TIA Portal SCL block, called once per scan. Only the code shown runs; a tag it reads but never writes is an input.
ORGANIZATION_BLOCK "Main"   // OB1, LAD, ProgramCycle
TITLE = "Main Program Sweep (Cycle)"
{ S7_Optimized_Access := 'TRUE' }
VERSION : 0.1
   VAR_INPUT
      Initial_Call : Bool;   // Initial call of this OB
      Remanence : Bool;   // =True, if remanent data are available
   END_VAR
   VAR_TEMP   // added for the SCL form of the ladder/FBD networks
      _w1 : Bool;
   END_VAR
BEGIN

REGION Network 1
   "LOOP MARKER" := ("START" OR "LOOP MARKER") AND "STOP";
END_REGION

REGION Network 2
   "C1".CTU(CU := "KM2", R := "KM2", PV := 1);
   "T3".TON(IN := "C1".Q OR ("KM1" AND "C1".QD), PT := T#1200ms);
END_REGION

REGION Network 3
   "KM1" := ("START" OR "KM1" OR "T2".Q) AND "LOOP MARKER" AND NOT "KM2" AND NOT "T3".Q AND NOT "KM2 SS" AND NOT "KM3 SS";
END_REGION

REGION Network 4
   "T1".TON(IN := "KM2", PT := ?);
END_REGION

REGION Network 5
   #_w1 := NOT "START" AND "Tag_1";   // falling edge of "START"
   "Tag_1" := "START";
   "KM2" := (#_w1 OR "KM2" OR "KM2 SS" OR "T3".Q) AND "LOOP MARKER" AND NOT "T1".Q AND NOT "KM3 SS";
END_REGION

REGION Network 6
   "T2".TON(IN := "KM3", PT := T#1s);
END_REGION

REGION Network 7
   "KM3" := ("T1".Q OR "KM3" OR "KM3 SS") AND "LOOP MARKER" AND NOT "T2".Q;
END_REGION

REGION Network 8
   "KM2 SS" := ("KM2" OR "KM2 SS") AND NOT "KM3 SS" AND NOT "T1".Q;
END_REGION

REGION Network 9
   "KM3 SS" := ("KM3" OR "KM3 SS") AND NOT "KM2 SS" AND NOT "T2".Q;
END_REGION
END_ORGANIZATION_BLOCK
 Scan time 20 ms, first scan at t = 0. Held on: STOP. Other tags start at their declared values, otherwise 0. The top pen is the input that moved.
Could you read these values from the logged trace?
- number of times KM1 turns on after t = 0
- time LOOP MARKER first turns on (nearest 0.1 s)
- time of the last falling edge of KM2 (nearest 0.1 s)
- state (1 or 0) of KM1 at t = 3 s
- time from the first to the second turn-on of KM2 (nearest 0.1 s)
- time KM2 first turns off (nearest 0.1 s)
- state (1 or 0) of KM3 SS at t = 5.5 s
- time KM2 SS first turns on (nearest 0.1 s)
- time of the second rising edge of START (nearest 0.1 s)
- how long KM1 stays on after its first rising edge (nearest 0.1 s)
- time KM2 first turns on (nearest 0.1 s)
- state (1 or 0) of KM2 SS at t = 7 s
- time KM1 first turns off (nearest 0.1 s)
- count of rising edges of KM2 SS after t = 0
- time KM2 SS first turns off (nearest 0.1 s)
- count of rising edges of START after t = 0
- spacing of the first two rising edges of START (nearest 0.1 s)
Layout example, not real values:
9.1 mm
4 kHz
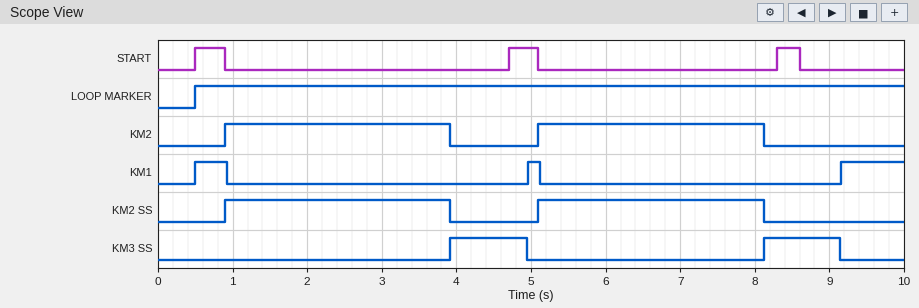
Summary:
3
0.5 s
8.1 s
0
4.2 s
3.9 s
0
0.9 s
4.7 s
0.4 s
0.9 s
1
0.9 s
2
3.9 s
3
4.2 s
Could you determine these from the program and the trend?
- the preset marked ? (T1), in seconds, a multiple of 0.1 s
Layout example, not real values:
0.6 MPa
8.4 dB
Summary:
3.0 s
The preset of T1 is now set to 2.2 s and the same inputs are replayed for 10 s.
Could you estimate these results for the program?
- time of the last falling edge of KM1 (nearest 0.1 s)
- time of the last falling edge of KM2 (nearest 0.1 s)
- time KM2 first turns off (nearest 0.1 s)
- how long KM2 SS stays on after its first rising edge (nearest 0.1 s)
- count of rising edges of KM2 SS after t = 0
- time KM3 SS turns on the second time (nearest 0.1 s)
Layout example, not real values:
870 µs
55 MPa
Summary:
8.6 s
7.3 s
3.1 s
2.2 s
3
7.3 s
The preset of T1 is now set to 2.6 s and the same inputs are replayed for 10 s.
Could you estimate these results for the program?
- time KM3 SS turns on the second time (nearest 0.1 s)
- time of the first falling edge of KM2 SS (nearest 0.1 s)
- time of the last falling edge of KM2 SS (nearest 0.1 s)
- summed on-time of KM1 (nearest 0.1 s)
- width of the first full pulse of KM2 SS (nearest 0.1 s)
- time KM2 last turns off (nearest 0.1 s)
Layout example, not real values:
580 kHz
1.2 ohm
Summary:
7.7 s
3.5 s
7.7 s
2.2 s
2.6 s
7.7 s
